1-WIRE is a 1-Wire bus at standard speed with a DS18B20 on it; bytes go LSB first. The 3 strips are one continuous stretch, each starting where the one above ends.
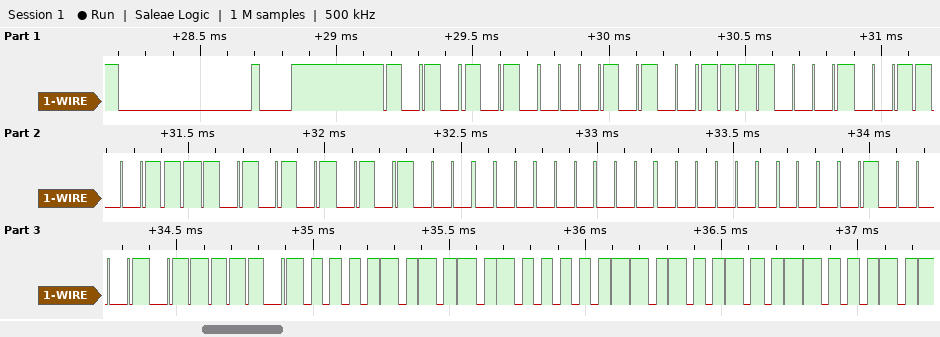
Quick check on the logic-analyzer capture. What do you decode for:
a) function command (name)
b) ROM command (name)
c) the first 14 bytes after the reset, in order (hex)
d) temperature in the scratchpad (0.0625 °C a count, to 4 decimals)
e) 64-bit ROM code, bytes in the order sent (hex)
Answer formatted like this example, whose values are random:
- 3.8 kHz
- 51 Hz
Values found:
- Read Scratchpad
- Match ROM
- 55 28 8F CC AB 0A 00 00 84 BE 50 05 4B 46
- 85.0000 °C
- 28 8F CC AB 0A 00 00 84
